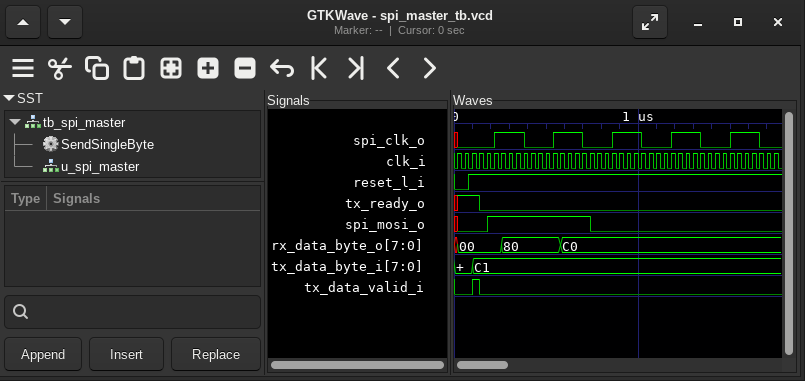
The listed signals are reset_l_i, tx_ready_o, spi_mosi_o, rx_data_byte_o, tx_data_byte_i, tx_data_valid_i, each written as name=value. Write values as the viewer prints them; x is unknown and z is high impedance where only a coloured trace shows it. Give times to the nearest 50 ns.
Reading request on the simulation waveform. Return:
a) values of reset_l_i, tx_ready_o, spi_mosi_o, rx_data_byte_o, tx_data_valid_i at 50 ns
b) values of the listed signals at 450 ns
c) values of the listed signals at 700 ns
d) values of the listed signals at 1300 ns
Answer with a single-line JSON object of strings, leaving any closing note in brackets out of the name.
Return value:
{"values of reset_l_i, tx_ready_o, spi_mosi_o, rx_data_byte_o, tx_data_valid_i at 50 ns": "reset_l_i=0, tx_ready_o=1, spi_mosi_o=0, rx_data_byte_o=00, tx_data_valid_i=0", "values of the listed signals at 450 ns": "reset_l_i=1, tx_ready_o=0, spi_mosi_o=1, rx_data_byte_o=80, tx_data_byte_i=C1, tx_data_valid_i=0", "values of the listed signals at 700 ns": "reset_l_i=1, tx_ready_o=0, spi_mosi_o=1, rx_data_byte_o=C0, tx_data_byte_i=C1, tx_data_valid_i=0", "values of the listed signals at 1300 ns": "reset_l_i=1, tx_ready_o=0, spi_mosi_o=0, rx_data_byte_o=C0, tx_data_byte_i=C1, tx_data_valid_i=0"}
